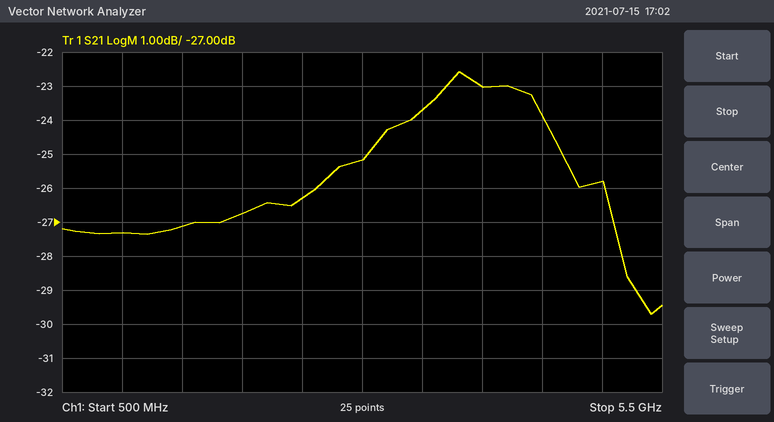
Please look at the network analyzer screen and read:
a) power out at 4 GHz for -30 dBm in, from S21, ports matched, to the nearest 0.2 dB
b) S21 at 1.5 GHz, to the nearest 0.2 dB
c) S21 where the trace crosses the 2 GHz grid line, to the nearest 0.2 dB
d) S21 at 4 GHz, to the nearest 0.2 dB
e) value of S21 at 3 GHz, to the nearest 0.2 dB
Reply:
-53.0 dBm
-27.2 dB
-26.8 dB
-23.0 dB
-25.2 dB
